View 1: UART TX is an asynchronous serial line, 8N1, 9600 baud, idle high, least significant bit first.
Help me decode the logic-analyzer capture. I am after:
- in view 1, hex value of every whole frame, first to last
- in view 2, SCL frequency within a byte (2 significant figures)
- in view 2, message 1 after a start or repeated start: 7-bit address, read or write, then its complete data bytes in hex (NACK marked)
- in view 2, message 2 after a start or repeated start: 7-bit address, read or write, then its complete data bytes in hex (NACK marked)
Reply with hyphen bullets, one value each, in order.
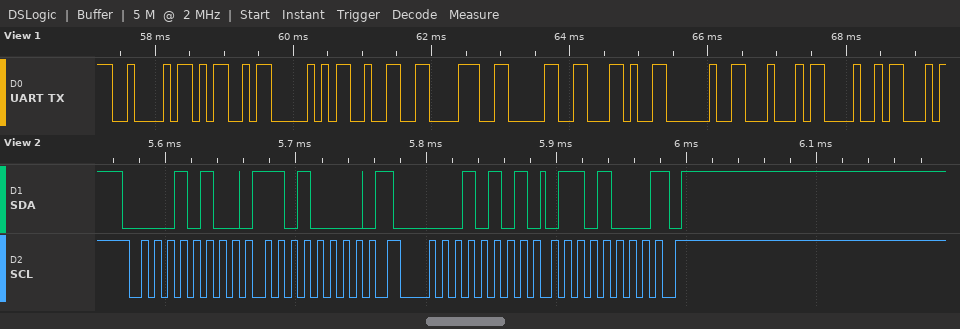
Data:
- 0x42 0x4D 0x50 0x32 0x38 0x30 0x2C 0x20 0x44 0x48
- 100 kHz
- 0x0A write: D0
- 0x0A read: 68 NACK
